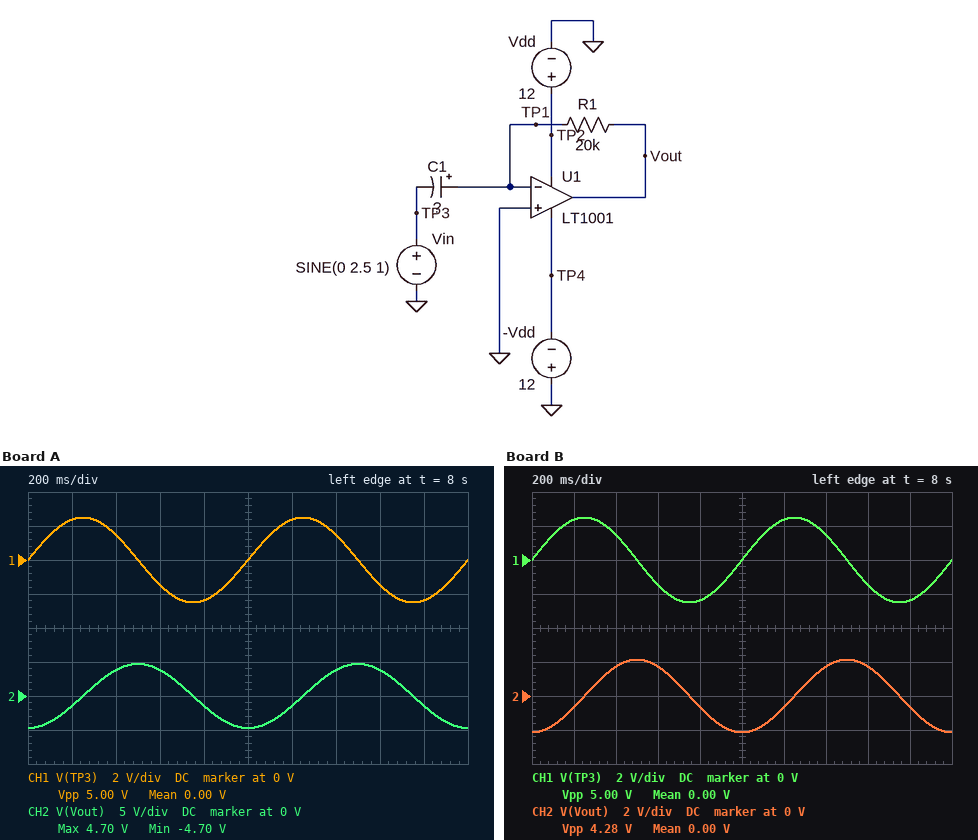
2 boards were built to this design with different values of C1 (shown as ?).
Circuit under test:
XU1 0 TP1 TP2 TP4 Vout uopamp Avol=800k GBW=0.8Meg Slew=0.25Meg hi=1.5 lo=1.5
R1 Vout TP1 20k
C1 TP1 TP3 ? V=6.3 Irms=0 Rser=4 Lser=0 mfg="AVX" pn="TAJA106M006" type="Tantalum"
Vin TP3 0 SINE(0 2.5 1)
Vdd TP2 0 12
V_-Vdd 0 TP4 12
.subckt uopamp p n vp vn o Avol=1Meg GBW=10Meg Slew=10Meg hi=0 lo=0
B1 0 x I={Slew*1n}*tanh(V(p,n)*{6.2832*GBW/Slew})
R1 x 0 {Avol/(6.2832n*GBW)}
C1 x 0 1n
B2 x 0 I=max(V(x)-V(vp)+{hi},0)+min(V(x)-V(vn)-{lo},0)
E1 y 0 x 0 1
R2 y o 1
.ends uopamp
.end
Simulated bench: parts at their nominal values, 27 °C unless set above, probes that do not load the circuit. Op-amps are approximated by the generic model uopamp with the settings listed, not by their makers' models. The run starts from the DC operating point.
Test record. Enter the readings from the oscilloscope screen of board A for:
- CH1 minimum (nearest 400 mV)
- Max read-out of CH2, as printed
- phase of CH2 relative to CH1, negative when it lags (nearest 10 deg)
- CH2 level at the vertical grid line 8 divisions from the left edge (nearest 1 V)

-2.4 V
4.70 V
-90 deg
4 V
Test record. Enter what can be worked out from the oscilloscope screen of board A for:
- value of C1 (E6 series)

15 µF
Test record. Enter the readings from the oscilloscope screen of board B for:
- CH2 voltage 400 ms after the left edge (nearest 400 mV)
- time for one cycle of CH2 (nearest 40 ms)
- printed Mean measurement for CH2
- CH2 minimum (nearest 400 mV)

1.6 V
1.00 s
0.00 V
-2.0 V
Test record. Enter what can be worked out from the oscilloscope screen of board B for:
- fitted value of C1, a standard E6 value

6.8 µF
